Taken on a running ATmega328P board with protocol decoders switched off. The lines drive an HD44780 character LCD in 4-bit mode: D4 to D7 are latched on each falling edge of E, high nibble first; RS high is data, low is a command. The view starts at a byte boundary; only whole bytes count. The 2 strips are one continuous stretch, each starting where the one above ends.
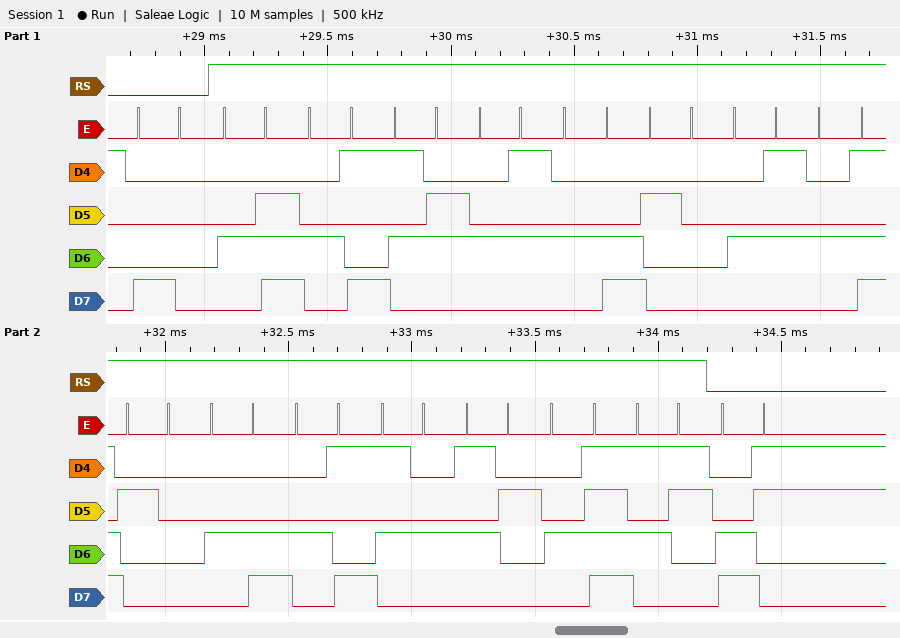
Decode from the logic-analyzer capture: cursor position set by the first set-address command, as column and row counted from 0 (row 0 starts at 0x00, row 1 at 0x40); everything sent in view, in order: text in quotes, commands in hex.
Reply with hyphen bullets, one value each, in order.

- column 0, row 0
- 0x80 "NIVEL EM LITROS" 0xC3
